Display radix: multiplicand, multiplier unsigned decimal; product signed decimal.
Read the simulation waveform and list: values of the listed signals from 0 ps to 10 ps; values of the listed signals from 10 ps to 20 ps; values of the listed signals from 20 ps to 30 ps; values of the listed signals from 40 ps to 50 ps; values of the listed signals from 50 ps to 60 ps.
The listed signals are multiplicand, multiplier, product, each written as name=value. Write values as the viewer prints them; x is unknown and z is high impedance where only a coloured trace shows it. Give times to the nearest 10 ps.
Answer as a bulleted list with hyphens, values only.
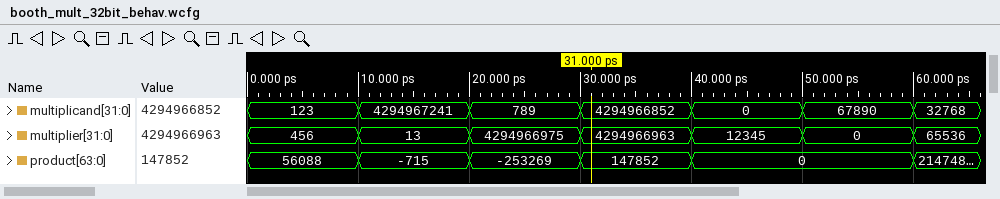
- multiplicand=123, multiplier=456, product=56088
- multiplicand=4294967241, multiplier=13, product=-715
- multiplicand=789, multiplier=4294966975, product=-253269
- multiplicand=0, multiplier=12345, product=0
- multiplicand=67890, multiplier=0, product=0
